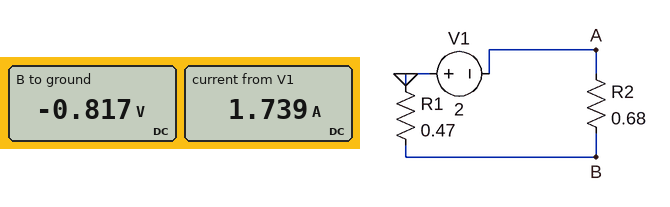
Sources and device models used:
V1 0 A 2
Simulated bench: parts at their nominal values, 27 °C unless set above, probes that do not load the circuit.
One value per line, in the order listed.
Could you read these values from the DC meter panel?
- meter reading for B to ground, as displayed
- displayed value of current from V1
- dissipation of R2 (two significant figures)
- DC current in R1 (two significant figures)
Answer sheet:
-0.817 V
1.739 A
2.1 W
1.7 A
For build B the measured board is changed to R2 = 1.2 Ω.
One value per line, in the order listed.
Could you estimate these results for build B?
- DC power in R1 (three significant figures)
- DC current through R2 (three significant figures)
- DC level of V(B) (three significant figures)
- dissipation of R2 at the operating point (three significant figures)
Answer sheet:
674 mW
1.20 A
-563 mV
1.72 W
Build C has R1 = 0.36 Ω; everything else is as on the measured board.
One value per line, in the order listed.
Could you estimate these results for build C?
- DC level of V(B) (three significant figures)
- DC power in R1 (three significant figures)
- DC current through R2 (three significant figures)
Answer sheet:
-692 mV
1.33 W
1.92 A
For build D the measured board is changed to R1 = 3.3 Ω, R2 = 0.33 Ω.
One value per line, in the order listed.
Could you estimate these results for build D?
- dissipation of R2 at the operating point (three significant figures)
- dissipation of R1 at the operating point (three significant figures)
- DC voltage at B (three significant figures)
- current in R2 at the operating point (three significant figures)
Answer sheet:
100 mW
1.00 W
-1.82 V
551 mA
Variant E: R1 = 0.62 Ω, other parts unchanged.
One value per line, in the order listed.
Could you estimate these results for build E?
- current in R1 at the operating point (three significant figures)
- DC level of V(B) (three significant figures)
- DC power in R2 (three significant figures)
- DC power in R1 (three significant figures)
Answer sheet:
1.54 A
-954 mV
1.61 W
1.47 W
